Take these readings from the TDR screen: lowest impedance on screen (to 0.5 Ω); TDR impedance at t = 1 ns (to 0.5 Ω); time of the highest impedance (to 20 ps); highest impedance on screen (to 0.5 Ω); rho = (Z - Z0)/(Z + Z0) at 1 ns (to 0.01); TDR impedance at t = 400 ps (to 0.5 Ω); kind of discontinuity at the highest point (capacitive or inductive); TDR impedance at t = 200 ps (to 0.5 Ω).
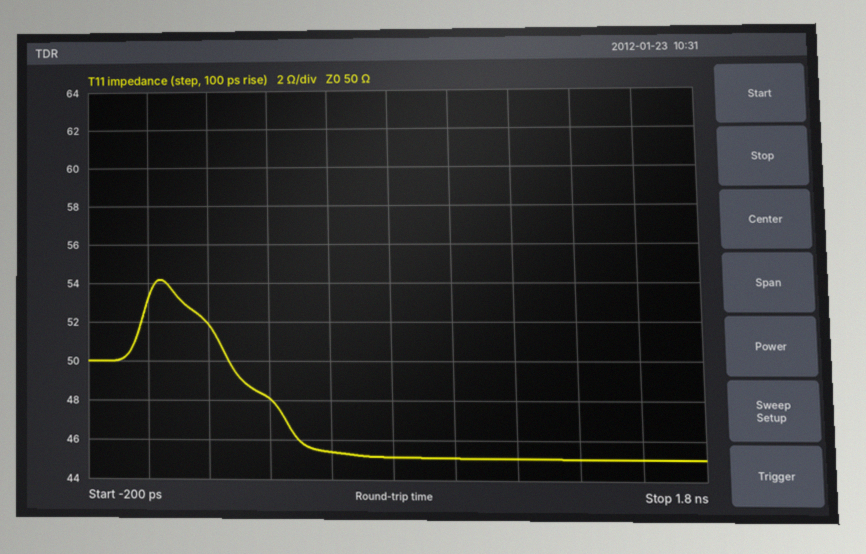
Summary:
45.0 Ω
45.0 Ω
40 ps
54.0 Ω
-0.05
48.0 Ω
inductive
52.0 Ω
